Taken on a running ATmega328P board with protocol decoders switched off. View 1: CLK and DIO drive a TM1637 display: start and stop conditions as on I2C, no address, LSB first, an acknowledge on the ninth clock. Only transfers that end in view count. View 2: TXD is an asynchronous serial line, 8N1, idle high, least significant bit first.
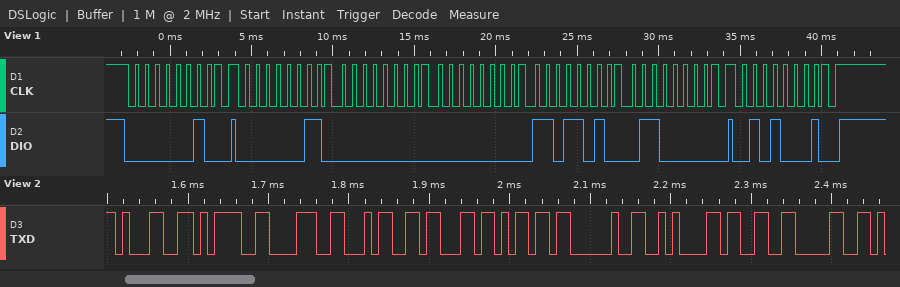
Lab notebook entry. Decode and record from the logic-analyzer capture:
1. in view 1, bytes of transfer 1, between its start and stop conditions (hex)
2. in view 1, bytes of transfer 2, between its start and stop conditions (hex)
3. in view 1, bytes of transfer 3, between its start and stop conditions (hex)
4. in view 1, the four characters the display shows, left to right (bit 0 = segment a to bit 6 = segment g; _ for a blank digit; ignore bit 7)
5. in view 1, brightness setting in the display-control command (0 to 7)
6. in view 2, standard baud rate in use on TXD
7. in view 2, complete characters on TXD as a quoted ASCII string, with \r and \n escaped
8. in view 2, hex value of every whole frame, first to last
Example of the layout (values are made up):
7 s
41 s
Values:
40
C0 00 00 5B 06
8A
__21
2
115200 baud
"1=84cm \n30"
0x31 0x3D 0x38 0x34 0x63 0x6D 0x20 0x0A 0x33 0x30
